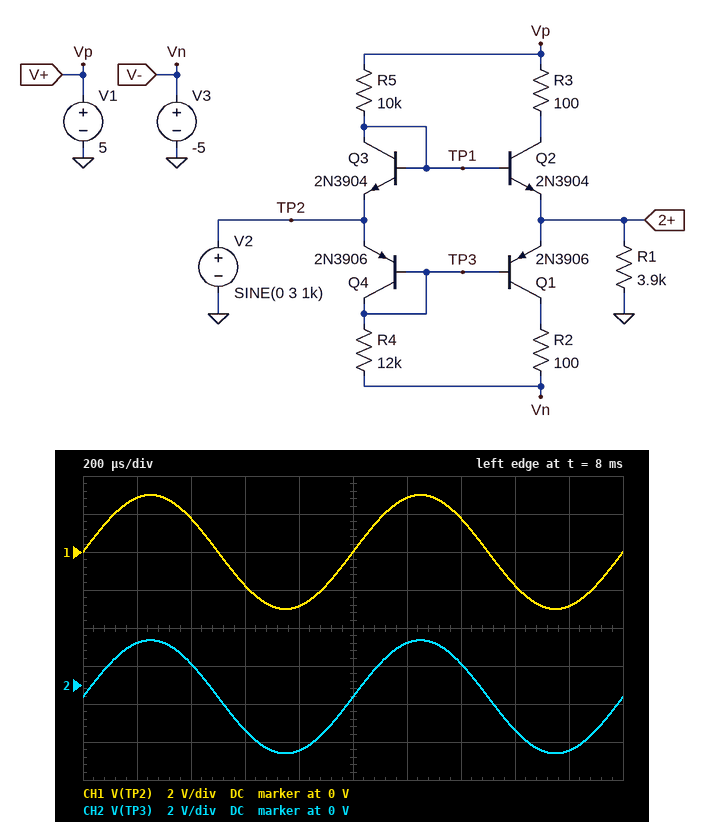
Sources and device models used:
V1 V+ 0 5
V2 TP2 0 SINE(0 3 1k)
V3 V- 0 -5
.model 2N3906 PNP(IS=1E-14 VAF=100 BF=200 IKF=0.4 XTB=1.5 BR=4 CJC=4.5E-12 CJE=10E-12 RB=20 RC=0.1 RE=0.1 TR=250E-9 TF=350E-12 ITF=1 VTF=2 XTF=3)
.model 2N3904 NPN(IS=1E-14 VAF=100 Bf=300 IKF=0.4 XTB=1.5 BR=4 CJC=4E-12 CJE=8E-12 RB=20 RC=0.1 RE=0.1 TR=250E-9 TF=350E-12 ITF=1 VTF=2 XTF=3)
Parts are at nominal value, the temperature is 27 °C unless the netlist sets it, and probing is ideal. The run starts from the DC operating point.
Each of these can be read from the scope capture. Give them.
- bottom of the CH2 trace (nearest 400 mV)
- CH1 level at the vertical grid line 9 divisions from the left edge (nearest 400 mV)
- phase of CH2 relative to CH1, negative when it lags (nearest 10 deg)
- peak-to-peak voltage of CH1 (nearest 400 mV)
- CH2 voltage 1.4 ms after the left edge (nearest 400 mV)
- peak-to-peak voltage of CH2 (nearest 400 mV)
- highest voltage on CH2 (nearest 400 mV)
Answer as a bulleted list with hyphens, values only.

- -3.6 V
- -2.8 V
- 0 deg
- 6.0 V
- 1.2 V
- 6.0 V
- 2.4 V
